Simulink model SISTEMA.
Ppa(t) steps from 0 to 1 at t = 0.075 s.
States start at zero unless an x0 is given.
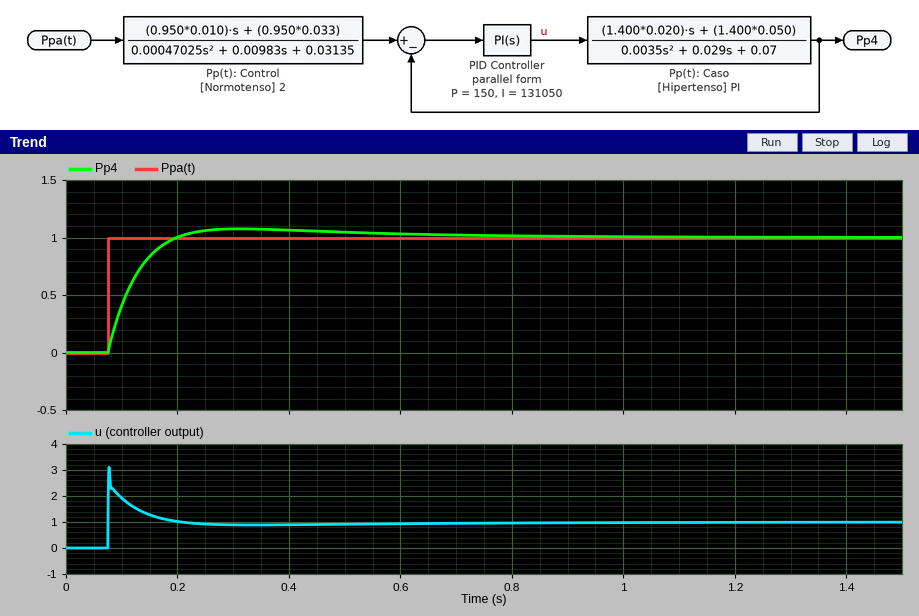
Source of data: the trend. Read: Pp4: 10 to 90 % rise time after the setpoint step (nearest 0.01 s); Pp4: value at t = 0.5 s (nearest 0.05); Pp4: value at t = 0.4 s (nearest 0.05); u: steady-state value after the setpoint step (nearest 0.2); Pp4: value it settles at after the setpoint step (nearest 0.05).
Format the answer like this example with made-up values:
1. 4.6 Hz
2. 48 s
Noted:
1. 0.08 s
2. 1.05
3. 1.05
4. 1.0
5. 1.00
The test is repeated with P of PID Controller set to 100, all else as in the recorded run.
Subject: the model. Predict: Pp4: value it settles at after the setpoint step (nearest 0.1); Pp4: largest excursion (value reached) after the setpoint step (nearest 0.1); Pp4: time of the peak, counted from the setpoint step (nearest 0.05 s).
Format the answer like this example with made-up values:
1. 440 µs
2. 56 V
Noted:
1. 1.0
2. 1.1
3. 0.25 s
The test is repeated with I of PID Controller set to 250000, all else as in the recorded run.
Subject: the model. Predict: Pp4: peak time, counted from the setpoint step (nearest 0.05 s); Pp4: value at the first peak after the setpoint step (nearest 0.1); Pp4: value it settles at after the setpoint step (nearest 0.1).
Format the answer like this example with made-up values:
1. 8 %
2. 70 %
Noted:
1. 0.25 s
2. 1.1
3. 1.0
